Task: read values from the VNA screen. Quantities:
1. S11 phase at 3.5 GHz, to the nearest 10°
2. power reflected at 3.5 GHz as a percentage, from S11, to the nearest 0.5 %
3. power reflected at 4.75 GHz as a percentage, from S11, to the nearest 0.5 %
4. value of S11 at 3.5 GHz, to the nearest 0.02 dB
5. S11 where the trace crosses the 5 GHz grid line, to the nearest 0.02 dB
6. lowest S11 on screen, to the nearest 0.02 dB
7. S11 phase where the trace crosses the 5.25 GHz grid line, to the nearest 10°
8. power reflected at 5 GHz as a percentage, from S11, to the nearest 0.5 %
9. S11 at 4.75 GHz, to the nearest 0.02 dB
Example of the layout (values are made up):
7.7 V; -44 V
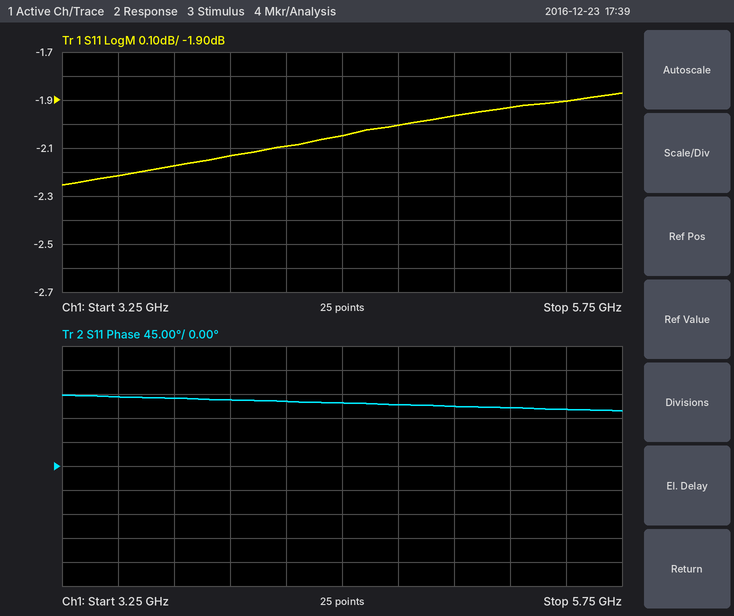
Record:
130°; 60.0 %; 63.0 %; -2.22 dB; -1.96 dB; -2.26 dB; 110°; 63.5 %; -2.00 dB
